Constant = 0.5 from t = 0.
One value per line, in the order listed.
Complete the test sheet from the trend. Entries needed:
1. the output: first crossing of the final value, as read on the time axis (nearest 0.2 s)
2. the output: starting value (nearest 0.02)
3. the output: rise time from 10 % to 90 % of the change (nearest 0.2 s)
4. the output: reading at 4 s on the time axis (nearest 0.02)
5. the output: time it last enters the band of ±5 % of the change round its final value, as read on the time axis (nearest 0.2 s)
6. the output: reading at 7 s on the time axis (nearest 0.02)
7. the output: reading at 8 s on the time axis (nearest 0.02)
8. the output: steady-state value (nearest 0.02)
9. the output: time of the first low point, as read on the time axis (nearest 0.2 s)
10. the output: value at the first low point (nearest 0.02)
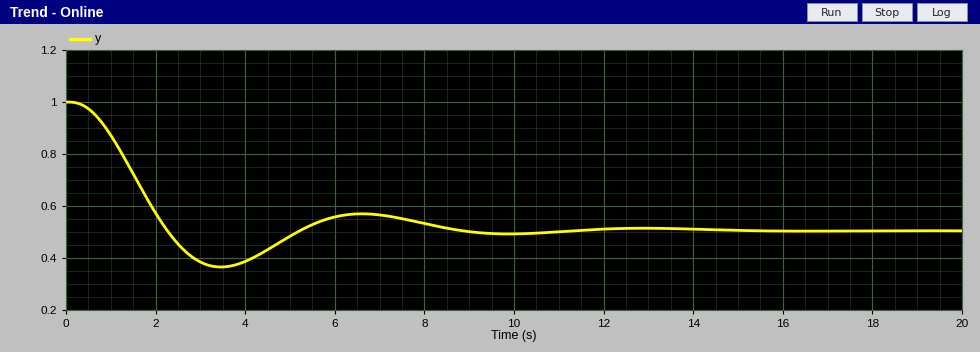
2.2 s
1.00
1.4 s
0.38
8.2 s
0.56
0.54
0.50
3.4 s
0.36
